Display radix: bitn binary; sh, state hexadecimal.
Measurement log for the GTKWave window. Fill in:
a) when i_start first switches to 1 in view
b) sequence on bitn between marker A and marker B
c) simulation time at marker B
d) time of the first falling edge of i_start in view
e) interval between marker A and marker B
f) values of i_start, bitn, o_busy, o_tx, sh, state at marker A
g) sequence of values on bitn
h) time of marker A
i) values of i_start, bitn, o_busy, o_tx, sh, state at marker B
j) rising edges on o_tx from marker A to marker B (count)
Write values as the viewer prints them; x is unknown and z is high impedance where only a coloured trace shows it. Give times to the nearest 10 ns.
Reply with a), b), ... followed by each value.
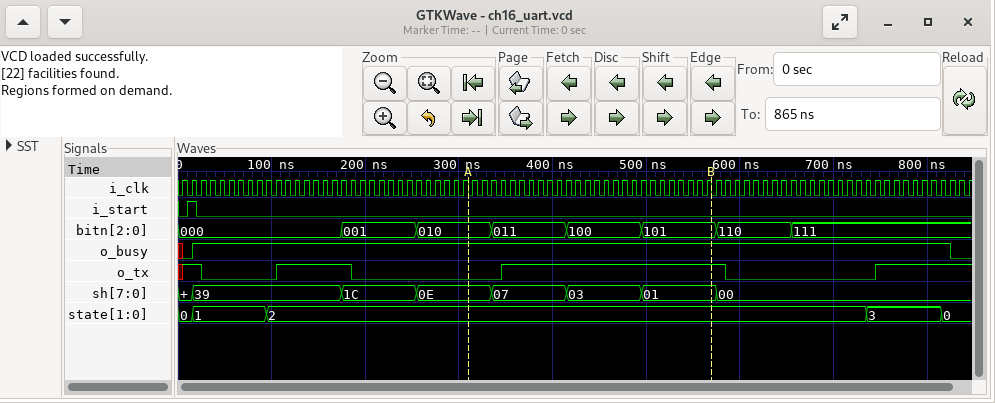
a) 10 ns
b) 010, 011, 100, 101
c) 570 ns
d) 20 ns
e) 260 ns
f) i_start=0, bitn=010, o_busy=1, o_tx=0, sh=0E, state=2
g) 000, 001, 010, 011, 100, 101, 110, 111
h) 310 ns
i) i_start=0, bitn=101, o_busy=1, o_tx=1, sh=01, state=2
j) 1
